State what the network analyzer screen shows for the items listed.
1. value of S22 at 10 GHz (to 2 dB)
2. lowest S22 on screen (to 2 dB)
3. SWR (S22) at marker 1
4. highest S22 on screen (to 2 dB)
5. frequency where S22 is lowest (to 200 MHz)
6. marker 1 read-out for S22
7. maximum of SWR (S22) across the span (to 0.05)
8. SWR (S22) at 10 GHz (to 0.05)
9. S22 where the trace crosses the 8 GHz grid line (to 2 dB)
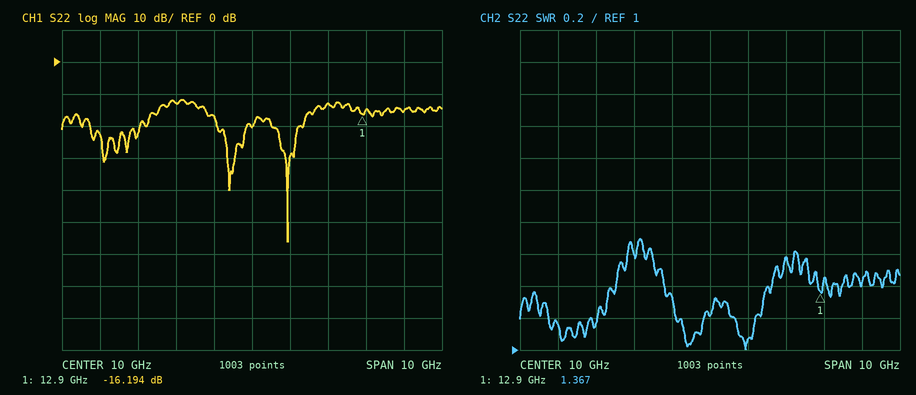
-20 dB
-56 dB
1.367
-12 dB
11.0 GHz
-16.194 dB
1.70
1.20
-12 dB
